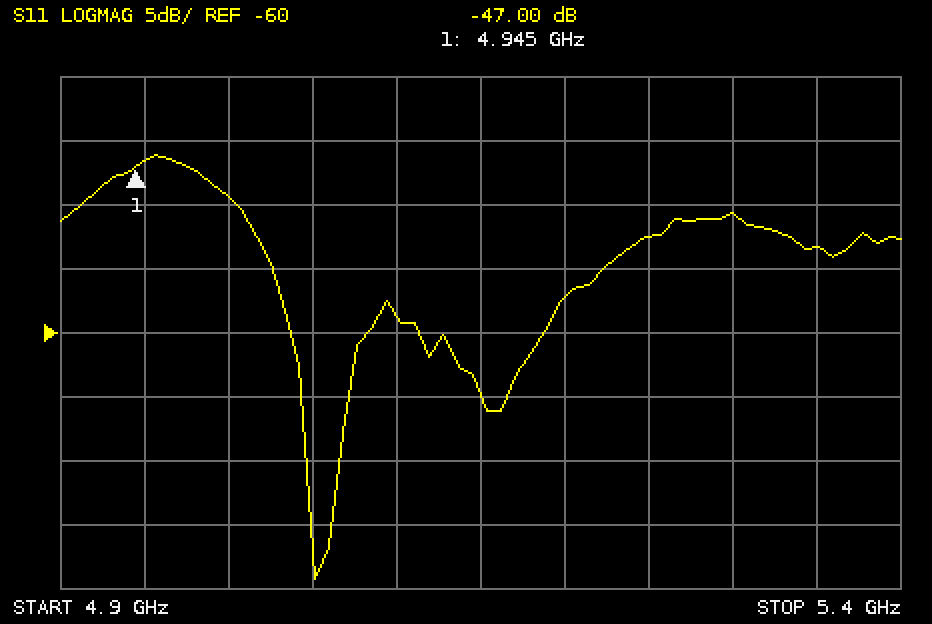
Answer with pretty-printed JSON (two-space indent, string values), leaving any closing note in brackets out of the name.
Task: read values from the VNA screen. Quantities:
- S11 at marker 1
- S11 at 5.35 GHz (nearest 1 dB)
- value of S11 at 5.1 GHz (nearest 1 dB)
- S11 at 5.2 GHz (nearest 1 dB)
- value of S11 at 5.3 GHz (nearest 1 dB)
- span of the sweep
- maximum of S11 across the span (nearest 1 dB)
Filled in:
{
  "S11 at marker 1": "-47.00 dB",
  "S11 at 5.35 GHz": "-53 dB",
  "value of S11 at 5.1 GHz": "-59 dB",
  "S11 at 5.2 GHz": "-57 dB",
  "value of S11 at 5.3 GHz": "-51 dB",
  "span of the sweep": "500 MHz",
  "maximum of S11 across the span": "-46 dB"
}
